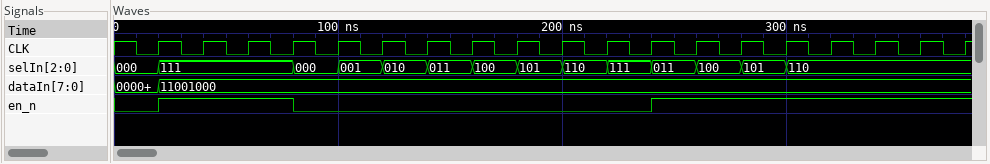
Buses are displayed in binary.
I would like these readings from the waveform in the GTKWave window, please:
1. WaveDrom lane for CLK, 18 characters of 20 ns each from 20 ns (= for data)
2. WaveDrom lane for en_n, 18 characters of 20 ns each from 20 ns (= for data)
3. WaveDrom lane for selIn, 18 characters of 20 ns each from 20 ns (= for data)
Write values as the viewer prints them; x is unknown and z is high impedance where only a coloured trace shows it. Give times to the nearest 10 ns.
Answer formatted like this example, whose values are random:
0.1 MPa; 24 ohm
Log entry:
{name: 'CLK', wave: 'p.................'}; {name: 'en_n', wave: '1..0.......1......'}; {name: 'selIn', wave: '=..============...', data: '111 000 001 010 011 100 101 110 111 011 100 101 110'}
